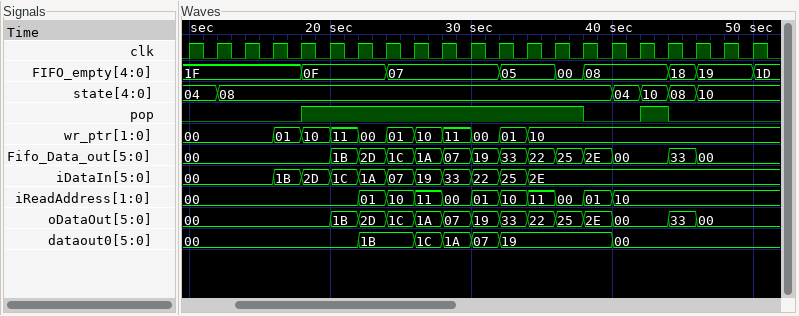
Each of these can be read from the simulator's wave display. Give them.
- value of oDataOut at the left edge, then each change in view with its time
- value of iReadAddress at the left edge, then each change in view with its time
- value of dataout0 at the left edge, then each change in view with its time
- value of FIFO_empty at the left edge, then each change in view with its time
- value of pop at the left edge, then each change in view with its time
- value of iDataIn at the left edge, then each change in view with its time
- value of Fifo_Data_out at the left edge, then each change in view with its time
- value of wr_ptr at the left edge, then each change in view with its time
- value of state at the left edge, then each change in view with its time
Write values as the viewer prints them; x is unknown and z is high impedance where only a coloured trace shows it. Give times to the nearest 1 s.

00, 1B at 20 s, 2D at 22 s, 1C at 24 s, 1A at 26 s, 07 at 28 s, 19 at 30 s, 33 at 32 s, 22 at 34 s, 25 at 36 s, 2E at 38 s, 00 at 40 s, 33 at 44 s, 00 at 46 s
00, 01 at 22 s, 10 at 24 s, 11 at 26 s, 00 at 28 s, 01 at 30 s, 10 at 32 s, 11 at 34 s, 00 at 36 s, 01 at 38 s, 10 at 40 s
00, 1B at 22 s, 1C at 26 s, 1A at 28 s, 07 at 30 s, 19 at 32 s, 00 at 40 s
1F, 0F at 18 s, 07 at 24 s, 05 at 32 s, 00 at 36 s, 08 at 38 s, 18 at 44 s, 19 at 46 s, 1D at 50 s
0, 1 at 18 s, 0 at 38 s, 1 at 42 s, 0 at 44 s
00, 1B at 16 s, 2D at 18 s, 1C at 20 s, 1A at 22 s, 07 at 24 s, 19 at 26 s, 33 at 28 s, 22 at 30 s, 25 at 32 s, 2E at 34 s
00, 1B at 20 s, 2D at 22 s, 1C at 24 s, 1A at 26 s, 07 at 28 s, 19 at 30 s, 33 at 32 s, 22 at 34 s, 25 at 36 s, 2E at 38 s, 00 at 40 s, 33 at 44 s, 00 at 46 s
00, 01 at 16 s, 10 at 18 s, 11 at 20 s, 00 at 22 s, 01 at 24 s, 10 at 26 s, 11 at 28 s, 00 at 30 s, 01 at 32 s, 10 at 34 s
04, 08 at 12 s, 04 at 40 s, 10 at 42 s, 08 at 44 s, 10 at 46 s
